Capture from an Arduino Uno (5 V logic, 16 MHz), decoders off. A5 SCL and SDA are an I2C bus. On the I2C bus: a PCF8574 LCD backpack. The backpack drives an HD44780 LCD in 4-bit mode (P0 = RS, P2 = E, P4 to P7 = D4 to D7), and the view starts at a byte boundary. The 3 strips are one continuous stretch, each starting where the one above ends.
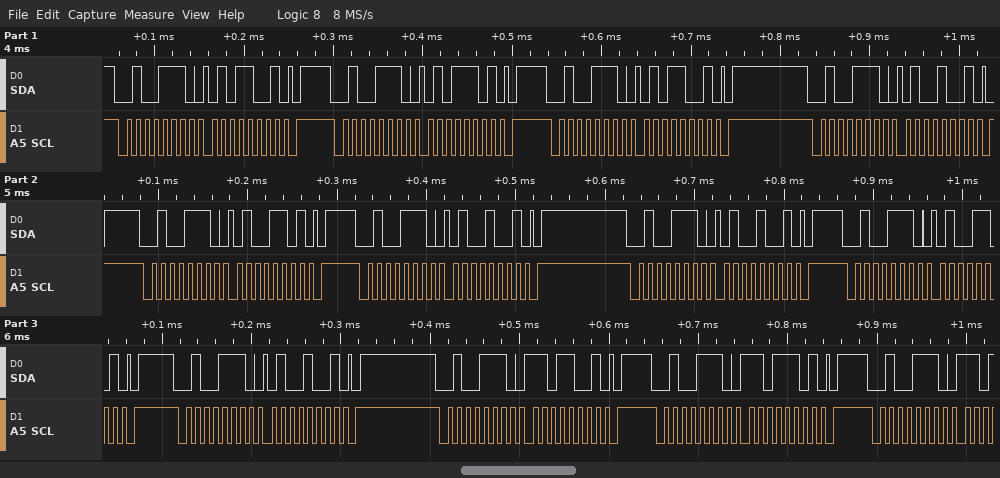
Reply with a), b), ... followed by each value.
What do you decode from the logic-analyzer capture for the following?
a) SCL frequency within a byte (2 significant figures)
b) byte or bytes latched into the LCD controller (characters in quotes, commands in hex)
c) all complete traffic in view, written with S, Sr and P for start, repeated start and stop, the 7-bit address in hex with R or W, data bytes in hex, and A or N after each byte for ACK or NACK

a) 100 kHz
b) 'T'
c) S 27W A 59 A P S 27W A 5D A P S 27W A 59 A P S 27W A 49 A P S 27W A 4D A P S 27W A 49 A P S 27W A 49 A P S 27W A 4D A P S 27W A 49 A P S 27W A D9 A P S 27W A DD A P S 27W A
